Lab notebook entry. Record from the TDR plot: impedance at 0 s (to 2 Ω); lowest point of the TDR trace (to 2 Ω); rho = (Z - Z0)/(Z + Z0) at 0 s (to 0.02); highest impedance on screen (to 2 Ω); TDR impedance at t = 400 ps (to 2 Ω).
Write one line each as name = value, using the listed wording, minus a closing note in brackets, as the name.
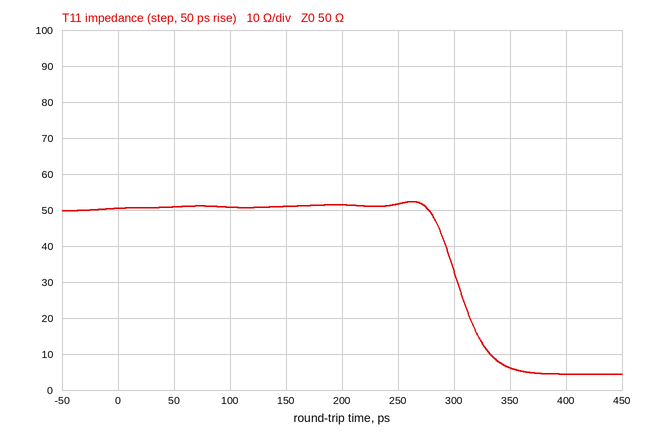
impedance at 0 s = 50 Ω
lowest point of the TDR trace = 4 Ω
rho = (Z - Z0)/(Z + Z0) at 0 s = 0.00
highest impedance on screen = 52 Ω
TDR impedance at t = 400 ps = 4 Ω
